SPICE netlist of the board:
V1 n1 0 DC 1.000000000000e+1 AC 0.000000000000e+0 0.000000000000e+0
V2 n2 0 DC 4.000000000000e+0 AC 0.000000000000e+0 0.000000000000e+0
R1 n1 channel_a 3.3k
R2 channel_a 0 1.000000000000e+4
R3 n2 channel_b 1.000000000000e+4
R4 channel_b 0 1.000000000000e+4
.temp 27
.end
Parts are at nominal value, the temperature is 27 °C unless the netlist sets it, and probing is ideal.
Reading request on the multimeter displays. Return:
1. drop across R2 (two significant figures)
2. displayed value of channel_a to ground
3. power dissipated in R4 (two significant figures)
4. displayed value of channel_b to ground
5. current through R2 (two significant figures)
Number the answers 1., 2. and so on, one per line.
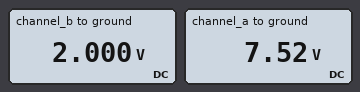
1. 7.5 V
2. 7.52 V
3. 400 µW
4. 2.000 V
5. 750 µA
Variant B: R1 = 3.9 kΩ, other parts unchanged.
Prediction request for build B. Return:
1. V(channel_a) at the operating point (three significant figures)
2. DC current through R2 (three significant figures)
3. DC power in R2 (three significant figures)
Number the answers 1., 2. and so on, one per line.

1. 7.19 V
2. 719 µA
3. 5.18 mW
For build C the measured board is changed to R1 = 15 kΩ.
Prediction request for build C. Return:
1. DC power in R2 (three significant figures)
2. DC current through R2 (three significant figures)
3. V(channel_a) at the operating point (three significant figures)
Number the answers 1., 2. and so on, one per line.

1. 1.60 mW
2. 400 µA
3. 4.00 V
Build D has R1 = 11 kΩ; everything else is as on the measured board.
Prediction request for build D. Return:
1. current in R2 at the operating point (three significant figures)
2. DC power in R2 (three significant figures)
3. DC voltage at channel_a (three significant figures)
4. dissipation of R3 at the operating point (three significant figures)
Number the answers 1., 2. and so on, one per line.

1. 476 µA
2. 2.27 mW
3. 4.76 V
4. 400 µW
